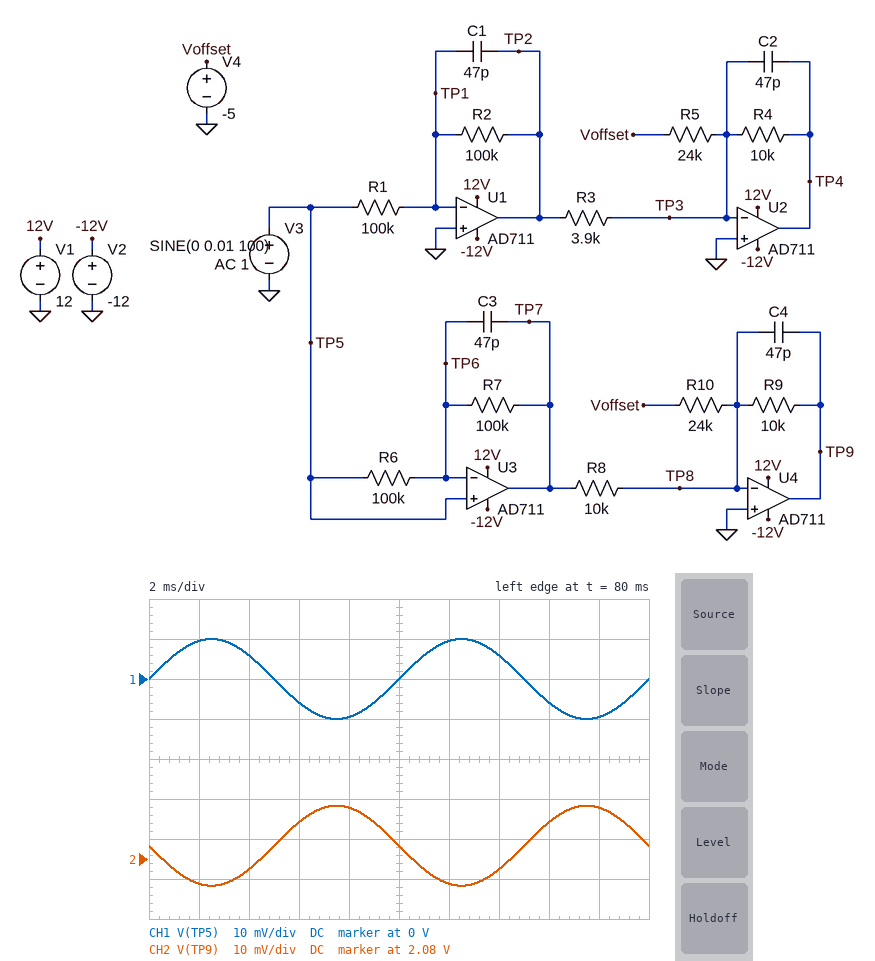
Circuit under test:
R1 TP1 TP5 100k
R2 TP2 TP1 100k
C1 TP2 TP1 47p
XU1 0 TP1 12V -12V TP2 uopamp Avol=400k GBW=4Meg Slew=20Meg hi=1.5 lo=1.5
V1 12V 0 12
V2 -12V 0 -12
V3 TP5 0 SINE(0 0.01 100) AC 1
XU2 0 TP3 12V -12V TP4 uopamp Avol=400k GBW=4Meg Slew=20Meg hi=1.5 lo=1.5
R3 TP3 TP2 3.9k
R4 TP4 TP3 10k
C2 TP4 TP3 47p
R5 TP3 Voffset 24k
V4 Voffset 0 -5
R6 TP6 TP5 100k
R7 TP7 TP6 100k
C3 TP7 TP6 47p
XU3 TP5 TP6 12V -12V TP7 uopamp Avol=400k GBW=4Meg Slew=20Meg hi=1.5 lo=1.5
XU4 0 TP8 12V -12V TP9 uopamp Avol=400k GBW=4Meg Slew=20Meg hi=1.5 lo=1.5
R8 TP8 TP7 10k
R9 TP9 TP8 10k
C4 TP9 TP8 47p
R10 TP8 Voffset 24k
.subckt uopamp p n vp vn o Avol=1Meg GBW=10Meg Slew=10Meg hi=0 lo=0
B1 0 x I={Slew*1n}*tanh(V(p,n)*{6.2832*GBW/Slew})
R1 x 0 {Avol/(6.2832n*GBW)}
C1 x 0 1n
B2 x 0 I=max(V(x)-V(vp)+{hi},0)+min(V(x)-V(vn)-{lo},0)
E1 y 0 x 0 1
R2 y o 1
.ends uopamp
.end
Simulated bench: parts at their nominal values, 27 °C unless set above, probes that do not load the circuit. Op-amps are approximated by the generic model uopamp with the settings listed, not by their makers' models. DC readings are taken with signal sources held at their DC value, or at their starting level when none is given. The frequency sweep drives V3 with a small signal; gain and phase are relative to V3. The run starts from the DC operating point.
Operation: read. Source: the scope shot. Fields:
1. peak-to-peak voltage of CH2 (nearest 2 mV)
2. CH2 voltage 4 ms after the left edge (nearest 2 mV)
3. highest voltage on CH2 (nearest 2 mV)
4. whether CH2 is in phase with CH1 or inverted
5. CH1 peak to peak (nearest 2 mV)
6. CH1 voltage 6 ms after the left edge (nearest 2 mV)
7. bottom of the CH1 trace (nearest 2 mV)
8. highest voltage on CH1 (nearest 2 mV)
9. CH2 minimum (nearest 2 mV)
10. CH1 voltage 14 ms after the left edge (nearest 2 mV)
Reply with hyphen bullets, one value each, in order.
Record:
- 20 mV
- 2.078 V
- 2.094 V
- inverted
- 20 mV
- -6 mV
- -10 mV
- 10 mV
- 2.074 V
- 6 mV
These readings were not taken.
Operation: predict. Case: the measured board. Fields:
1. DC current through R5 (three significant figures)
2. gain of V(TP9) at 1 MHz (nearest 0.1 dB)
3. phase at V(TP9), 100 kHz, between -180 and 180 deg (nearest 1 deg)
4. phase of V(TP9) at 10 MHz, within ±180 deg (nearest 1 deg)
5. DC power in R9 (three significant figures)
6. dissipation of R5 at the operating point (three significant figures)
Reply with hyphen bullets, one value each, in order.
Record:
- 208 µA
- -11.4 dB
- 159 deg
- -42 deg
- 434 µW
- 1.04 mW
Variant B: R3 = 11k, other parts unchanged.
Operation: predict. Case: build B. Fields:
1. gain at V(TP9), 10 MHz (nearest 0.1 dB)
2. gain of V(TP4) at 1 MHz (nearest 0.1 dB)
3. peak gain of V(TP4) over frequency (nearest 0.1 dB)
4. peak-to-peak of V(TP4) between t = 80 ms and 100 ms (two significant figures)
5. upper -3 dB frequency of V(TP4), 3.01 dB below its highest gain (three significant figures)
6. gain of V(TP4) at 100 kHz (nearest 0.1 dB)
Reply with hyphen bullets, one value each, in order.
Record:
- -46.7 dB
- -41.6 dB
- -0.8 dB
- 18 mV
- 33.2 kHz
- -11.2 dB
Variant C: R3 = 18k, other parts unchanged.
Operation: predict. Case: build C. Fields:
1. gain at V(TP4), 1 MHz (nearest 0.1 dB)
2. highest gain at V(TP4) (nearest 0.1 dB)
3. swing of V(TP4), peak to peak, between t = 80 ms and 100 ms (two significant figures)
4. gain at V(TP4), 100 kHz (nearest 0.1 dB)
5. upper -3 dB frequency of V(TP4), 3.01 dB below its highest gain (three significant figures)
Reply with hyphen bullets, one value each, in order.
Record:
- -45.6 dB
- -5.1 dB
- 11 mV
- -15.5 dB
- 33.2 kHz
